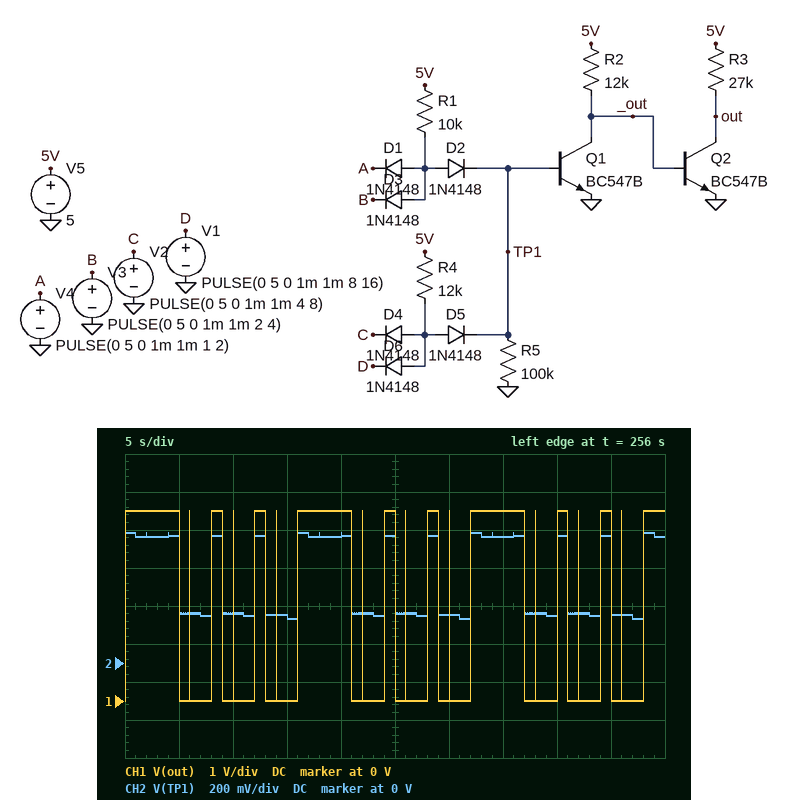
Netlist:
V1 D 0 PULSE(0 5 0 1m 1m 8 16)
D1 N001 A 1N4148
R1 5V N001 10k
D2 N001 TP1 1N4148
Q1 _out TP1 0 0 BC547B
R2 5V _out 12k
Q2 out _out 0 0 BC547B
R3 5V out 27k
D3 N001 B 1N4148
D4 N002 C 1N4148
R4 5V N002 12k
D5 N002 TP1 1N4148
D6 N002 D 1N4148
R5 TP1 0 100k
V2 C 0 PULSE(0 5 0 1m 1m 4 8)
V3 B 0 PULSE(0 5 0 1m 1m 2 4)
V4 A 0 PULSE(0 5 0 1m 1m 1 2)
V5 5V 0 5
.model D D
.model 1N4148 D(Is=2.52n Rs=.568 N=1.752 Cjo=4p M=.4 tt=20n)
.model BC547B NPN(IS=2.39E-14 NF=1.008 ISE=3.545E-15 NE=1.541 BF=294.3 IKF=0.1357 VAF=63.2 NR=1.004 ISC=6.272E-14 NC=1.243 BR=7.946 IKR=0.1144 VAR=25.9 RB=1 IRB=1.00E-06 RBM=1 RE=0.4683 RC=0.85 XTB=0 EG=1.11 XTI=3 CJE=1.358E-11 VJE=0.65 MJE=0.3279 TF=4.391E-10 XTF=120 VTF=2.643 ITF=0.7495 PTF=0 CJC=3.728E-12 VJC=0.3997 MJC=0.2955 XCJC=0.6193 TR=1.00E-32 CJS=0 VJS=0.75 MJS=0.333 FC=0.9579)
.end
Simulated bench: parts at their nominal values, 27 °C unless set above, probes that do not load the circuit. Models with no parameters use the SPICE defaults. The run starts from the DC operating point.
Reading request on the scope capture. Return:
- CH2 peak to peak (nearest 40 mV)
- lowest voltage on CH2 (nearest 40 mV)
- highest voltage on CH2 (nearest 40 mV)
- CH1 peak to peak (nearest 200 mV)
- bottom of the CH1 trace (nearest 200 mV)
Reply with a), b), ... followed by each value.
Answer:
a) 440 mV
b) 240 mV
c) 680 mV
d) 5.0 V
e) 0 V
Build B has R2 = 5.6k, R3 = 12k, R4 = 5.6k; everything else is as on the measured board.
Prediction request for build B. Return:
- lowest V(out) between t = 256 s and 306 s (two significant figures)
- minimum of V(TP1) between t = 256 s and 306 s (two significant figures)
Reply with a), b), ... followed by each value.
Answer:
a) 9.5 mV
b) 250 mV
